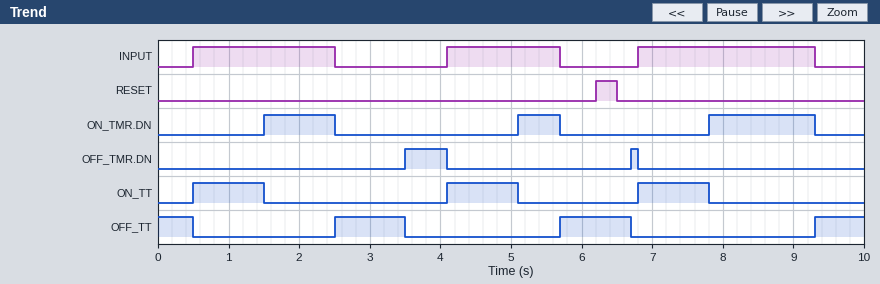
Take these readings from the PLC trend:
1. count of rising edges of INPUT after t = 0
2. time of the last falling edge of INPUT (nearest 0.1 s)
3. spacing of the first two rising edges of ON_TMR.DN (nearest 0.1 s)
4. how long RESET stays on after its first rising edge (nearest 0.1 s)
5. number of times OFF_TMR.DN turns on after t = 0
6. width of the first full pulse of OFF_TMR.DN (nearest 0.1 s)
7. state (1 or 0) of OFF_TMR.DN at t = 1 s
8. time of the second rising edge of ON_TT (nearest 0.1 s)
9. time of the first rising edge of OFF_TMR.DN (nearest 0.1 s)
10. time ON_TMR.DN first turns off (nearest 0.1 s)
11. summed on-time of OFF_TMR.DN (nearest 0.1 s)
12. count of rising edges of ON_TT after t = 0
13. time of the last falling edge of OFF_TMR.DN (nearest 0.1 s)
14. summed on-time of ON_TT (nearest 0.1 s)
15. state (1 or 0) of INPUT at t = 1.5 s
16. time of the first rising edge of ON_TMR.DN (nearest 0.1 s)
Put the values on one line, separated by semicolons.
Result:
3; 9.3 s; 3.6 s; 0.3 s; 2; 0.6 s; 0; 4.1 s; 3.5 s; 2.5 s; 0.7 s; 3; 6.8 s; 3.0 s; 1; 1.5 s
